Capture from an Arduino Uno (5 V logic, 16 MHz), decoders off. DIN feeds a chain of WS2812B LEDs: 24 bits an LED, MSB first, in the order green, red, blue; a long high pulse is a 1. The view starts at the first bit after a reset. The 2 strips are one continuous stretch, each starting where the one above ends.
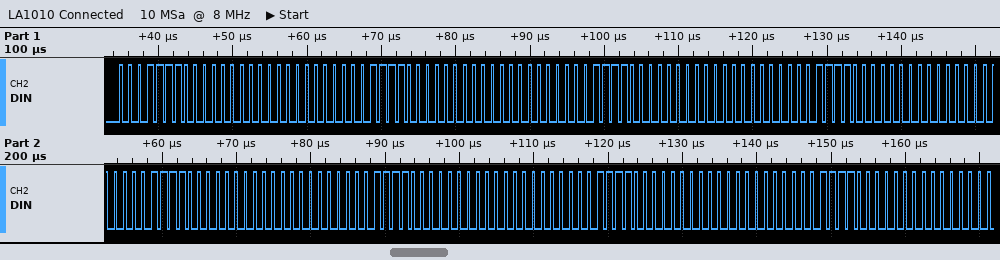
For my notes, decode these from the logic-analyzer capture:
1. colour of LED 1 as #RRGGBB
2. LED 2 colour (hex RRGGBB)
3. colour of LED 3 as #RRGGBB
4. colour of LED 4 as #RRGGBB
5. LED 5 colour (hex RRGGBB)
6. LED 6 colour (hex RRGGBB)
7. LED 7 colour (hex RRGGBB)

#001E00
#001E00
#001E00
#001E00
#001E00
#001E00
#001E00
